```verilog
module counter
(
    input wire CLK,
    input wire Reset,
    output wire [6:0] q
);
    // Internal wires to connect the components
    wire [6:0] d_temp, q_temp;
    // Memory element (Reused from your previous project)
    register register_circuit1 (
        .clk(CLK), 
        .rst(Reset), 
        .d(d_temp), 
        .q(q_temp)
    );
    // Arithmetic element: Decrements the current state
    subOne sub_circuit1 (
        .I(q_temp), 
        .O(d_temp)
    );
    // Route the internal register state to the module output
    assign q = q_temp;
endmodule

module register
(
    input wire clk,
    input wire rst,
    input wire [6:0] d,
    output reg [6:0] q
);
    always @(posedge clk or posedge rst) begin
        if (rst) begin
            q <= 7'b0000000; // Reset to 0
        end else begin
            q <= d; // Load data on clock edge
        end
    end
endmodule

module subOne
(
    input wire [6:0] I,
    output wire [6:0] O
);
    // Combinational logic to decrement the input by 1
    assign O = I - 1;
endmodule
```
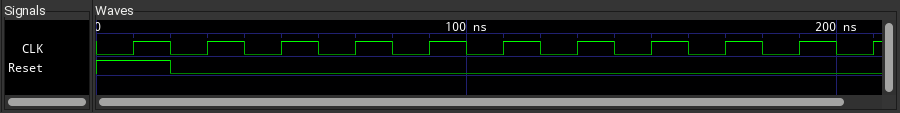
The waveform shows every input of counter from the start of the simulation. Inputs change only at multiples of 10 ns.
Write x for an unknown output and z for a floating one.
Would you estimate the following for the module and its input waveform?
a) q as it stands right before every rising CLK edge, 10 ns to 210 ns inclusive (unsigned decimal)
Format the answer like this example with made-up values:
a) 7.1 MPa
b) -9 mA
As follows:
a) 0, 0, 127, 126, 125, 124, 123, 122, 121, 120, 119
